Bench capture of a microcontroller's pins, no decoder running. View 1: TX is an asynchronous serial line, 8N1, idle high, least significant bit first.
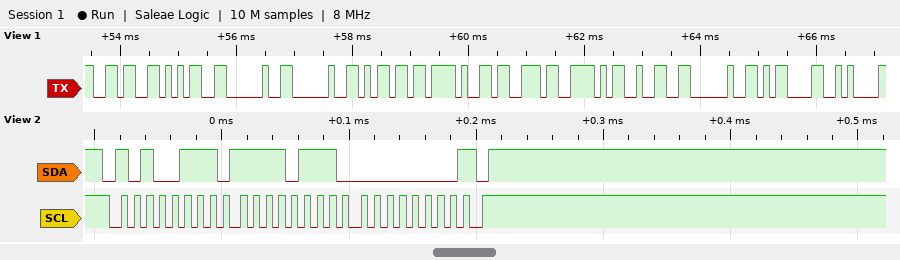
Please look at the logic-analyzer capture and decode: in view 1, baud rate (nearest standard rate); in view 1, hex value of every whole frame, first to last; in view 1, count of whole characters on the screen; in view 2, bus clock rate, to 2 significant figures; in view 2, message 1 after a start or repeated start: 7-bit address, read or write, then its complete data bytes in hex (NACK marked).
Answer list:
9600 baud
36 35 20 20 6D 2F 73 5E 32 20 0D 0A
12
100 kHz
0x53 read: F7 00 NACK
